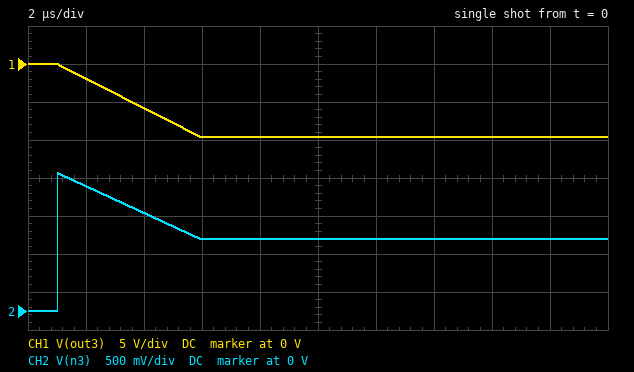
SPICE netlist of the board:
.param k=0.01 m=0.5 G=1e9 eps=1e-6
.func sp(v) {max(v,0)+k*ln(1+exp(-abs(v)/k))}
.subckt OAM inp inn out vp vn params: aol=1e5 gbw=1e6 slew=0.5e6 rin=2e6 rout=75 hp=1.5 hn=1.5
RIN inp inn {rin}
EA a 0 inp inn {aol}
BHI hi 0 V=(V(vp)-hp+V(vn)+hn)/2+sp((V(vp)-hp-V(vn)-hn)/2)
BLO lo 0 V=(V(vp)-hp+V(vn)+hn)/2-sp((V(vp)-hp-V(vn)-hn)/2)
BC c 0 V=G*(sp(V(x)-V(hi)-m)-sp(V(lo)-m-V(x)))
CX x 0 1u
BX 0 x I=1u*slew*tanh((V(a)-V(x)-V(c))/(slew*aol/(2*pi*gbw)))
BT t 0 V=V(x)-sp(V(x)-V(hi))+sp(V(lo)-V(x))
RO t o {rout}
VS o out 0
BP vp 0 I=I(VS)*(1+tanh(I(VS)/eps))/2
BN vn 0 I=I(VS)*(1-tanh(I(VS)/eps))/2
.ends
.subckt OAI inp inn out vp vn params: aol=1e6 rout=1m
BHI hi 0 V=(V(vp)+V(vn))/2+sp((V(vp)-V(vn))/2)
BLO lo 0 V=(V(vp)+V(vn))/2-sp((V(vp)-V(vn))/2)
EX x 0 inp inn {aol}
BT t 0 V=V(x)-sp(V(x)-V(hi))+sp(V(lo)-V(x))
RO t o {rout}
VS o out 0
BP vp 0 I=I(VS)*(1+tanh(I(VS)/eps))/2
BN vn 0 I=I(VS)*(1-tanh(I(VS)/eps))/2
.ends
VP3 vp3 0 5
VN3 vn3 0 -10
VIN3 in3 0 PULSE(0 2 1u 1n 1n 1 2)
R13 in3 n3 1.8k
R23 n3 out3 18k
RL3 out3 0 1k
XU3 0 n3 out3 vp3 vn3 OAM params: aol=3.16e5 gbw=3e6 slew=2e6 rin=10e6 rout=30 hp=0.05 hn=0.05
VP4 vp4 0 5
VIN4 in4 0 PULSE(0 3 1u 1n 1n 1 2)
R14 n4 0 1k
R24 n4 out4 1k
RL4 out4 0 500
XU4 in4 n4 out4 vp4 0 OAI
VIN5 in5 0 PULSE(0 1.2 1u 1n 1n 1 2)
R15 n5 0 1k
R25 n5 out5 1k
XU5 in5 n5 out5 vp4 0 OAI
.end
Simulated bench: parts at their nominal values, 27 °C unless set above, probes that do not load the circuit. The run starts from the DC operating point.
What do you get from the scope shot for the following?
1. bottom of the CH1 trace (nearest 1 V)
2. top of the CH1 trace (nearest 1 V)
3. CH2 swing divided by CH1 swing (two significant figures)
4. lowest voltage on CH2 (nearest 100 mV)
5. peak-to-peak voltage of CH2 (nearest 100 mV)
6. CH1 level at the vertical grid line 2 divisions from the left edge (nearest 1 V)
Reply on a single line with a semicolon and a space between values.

-10 V; 0 V; 0.19; 0 V; 1.8 V; -6 V
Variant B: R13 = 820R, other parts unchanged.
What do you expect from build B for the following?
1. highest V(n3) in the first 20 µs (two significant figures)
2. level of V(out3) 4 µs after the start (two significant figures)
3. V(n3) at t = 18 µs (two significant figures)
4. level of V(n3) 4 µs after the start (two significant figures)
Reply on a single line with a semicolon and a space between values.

1.9 V; -5.8 V; 1.5 V; 1.7 V
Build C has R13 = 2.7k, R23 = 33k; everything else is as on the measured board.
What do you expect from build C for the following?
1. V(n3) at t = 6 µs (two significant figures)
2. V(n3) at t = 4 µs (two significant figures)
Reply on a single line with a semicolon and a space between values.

1.1 V; 1.4 V
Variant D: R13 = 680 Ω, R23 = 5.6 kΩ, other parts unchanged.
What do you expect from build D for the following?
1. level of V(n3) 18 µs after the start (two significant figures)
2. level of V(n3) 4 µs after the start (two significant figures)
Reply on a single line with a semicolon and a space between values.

740 mV; 1.2 V
